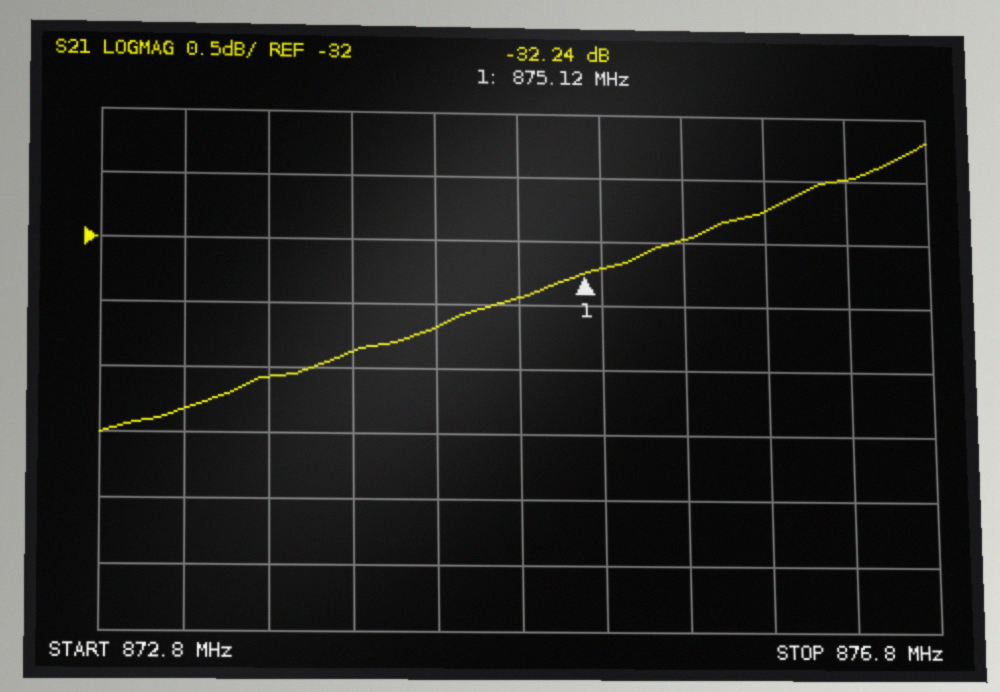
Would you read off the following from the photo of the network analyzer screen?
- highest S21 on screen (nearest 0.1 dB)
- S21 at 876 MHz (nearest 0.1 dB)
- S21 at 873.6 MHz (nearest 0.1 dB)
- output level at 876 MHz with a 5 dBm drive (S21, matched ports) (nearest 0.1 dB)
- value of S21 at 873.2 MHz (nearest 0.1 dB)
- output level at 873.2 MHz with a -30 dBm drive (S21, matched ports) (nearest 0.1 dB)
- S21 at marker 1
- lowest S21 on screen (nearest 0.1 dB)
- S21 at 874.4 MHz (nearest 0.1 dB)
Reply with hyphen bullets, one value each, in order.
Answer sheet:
- -31.2 dB
- -31.7 dB
- -33.1 dB
- -26.7 dBm
- -33.3 dB
- -63.3 dBm
- -32.24 dB
- -33.5 dB
- -32.7 dB
